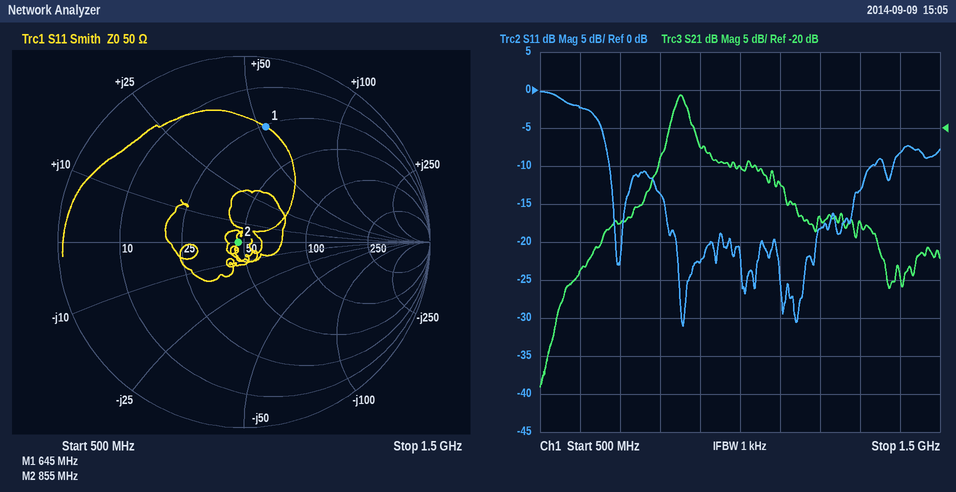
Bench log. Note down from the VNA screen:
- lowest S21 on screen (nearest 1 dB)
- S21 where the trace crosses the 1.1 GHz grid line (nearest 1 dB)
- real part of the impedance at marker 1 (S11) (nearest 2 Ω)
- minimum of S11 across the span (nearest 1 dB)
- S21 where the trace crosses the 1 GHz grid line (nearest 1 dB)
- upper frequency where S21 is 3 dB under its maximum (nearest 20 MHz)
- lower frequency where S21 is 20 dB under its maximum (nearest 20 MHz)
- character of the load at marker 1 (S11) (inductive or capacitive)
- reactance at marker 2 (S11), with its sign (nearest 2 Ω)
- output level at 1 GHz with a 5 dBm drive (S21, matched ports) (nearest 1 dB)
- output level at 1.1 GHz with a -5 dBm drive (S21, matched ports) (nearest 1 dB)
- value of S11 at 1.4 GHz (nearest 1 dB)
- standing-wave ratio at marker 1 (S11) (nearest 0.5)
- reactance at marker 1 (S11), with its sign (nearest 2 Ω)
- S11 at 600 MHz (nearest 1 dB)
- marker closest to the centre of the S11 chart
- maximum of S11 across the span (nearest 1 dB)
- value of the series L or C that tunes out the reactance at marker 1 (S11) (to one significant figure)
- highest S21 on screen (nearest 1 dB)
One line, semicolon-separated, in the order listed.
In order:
-54 dB; -27 dB; 26 Ω; -31 dB; -25 dB; 880 MHz; 640 MHz; inductive; 0 Ω; -20 dBm; -32 dBm; -8 dB; 4.5; +54 Ω; -2 dB; marker 2; 0 dB; 5 pF; -16 dB
